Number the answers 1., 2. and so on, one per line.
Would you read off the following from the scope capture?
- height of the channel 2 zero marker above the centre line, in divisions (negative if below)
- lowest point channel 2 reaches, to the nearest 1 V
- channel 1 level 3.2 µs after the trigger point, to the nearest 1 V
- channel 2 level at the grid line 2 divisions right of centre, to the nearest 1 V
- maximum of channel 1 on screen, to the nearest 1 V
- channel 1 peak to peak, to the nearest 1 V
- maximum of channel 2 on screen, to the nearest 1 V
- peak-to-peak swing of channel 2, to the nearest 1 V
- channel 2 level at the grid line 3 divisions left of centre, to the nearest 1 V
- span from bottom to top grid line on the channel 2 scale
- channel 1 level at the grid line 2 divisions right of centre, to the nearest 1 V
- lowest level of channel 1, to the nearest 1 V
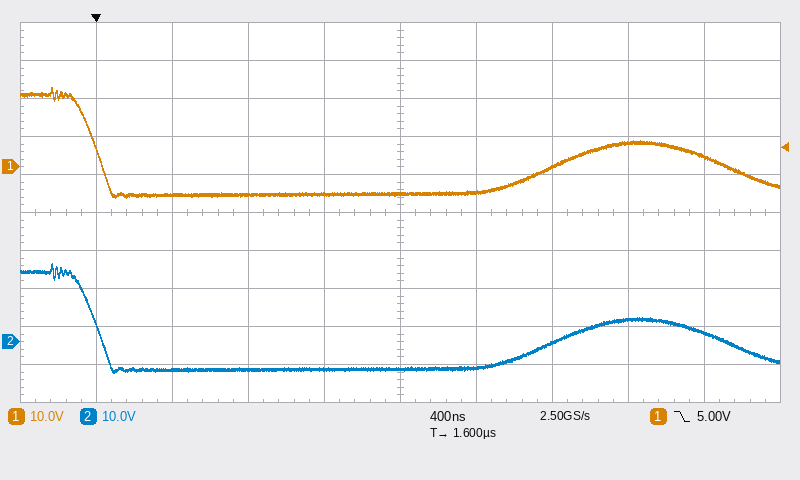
1. -3.4 div
2. -8 V
3. 3 V
4. 0 V
5. 21 V
6. 29 V
7. 21 V
8. 29 V
9. -7 V
10. 100 V
11. 0 V
12. -8 V
